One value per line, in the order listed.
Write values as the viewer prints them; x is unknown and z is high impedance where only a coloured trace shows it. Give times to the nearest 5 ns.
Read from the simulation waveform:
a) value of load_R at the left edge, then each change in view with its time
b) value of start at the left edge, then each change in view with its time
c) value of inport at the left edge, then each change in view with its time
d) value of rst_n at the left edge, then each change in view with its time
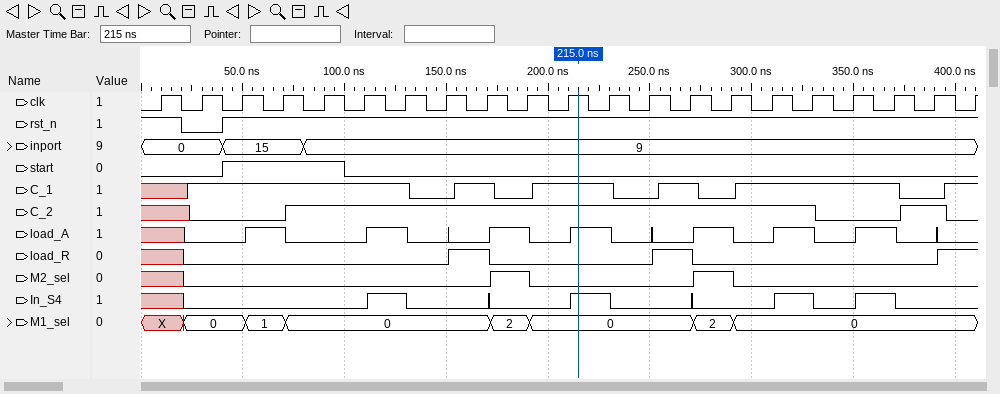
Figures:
x, 0 at 20 ns, 1 at 150 ns, 0 at 170 ns, 1 at 250 ns, 0 at 270 ns, 1 at 390 ns
0, 1 at 40 ns, 0 at 100 ns
0, 15 at 40 ns, 9 at 80 ns
1, 0 at 20 ns, 1 at 40 ns
